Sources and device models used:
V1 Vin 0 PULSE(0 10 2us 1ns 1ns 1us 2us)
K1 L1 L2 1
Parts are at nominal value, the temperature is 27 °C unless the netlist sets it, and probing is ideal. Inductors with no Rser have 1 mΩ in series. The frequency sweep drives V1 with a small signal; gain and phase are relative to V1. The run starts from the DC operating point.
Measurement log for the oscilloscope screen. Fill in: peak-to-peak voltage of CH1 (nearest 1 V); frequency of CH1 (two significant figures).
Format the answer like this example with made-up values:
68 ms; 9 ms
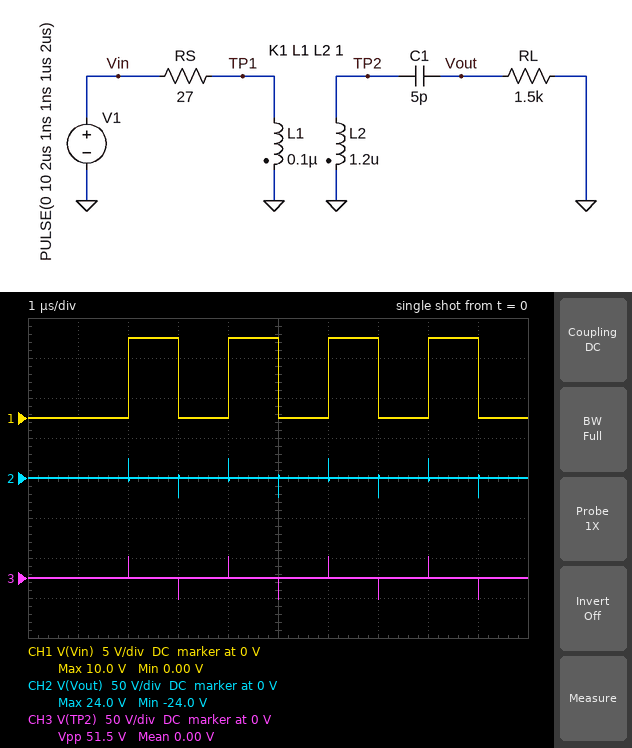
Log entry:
10 V; 500 kHz
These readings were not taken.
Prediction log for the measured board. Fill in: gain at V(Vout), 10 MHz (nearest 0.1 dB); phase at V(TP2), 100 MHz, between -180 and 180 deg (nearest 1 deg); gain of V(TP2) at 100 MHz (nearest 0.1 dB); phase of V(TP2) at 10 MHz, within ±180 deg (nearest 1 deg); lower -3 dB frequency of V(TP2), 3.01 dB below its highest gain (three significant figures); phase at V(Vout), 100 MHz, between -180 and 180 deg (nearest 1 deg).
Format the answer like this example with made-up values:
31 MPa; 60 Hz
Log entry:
-9.4 dB; 18 deg; 8.7 dB; 76 deg; 31.1 MHz; 30 deg
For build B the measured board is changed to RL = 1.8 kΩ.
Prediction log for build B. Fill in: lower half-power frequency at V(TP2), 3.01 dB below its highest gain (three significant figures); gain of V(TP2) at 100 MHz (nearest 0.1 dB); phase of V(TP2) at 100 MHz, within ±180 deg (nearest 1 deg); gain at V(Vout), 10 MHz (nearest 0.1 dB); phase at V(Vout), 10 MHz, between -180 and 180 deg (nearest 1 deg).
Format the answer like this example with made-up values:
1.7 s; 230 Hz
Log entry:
33.2 MHz; 8.9 dB; 19 deg; -8.1 dB; 137 deg
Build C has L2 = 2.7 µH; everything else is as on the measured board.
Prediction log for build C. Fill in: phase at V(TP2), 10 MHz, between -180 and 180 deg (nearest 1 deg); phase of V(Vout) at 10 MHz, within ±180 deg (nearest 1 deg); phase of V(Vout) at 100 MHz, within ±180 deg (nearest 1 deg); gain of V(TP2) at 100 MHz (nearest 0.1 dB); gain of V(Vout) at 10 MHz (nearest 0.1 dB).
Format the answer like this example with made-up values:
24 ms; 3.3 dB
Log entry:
75 deg; 140 deg; 25 deg; 10.8 dB; -5.7 dB
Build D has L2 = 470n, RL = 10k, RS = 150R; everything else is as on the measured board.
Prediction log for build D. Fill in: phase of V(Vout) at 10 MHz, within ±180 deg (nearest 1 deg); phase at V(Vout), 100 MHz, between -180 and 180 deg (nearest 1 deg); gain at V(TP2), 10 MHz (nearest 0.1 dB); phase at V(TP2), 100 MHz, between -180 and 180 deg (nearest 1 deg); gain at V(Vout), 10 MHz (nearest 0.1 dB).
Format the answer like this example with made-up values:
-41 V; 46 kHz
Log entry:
105 deg; 68 deg; -20.8 dB; 66 deg; -21.3 dB
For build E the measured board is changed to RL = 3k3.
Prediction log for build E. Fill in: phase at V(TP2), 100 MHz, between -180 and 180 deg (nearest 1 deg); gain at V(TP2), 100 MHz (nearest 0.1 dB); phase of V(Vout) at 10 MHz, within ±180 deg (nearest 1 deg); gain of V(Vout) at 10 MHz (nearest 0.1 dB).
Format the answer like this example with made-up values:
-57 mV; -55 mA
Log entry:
21 deg; 9.4 dB; 120 deg; -4.9 dB
